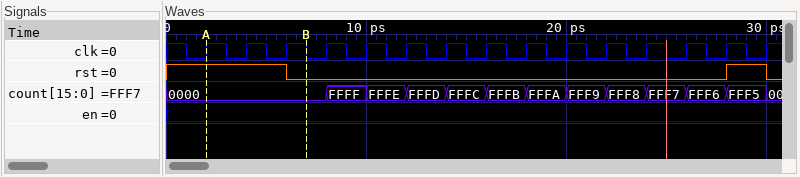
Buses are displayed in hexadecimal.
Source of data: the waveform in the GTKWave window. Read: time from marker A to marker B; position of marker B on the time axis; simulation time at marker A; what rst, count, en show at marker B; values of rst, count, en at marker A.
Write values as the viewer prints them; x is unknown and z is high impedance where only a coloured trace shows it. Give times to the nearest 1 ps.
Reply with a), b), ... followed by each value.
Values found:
a) 5 ps
b) 7 ps
c) 2 ps
d) rst=0, count=0000, en=0
e) rst=1, count=0000, en=0
